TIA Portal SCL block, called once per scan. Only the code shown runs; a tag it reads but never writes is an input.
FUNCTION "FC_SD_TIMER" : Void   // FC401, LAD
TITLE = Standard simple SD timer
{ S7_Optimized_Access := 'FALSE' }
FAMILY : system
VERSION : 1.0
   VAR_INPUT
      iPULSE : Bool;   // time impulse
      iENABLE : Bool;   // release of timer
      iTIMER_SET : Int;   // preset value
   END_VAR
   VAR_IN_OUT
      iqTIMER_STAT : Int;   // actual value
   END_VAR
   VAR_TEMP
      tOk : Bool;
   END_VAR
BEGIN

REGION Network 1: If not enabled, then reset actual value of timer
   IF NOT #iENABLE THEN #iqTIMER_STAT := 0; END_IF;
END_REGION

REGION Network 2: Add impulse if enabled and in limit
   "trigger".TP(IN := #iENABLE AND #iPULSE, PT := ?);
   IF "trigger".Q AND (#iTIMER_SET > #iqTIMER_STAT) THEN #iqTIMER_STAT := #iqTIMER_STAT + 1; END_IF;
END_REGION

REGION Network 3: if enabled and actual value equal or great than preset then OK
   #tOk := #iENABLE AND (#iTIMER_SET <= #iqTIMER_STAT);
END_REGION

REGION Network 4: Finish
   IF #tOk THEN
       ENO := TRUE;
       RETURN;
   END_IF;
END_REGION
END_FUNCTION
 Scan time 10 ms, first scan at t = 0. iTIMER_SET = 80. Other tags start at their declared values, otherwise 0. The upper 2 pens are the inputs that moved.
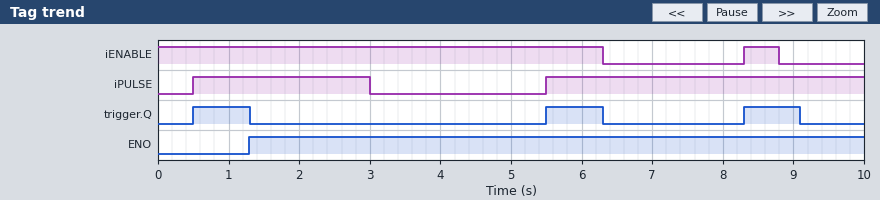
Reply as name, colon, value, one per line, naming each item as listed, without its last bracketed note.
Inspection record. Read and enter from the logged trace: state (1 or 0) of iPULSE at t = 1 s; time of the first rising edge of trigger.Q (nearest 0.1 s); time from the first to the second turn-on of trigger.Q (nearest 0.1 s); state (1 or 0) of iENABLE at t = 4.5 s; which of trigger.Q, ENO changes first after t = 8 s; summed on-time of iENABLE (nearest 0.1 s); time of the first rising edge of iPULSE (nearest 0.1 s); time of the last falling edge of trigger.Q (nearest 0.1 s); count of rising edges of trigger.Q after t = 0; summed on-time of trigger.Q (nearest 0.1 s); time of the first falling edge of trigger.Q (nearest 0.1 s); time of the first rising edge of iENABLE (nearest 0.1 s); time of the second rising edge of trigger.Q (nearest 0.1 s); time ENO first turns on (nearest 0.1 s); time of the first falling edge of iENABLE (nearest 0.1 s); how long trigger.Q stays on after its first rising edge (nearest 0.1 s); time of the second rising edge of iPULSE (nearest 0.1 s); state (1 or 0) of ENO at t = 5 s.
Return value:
state (1 or 0) of iPULSE at t = 1 s: 1
time of the first rising edge of trigger.Q: 0.5 s
time from the first to the second turn-on of trigger.Q: 5.0 s
state (1 or 0) of iENABLE at t = 4.5 s: 1
which of trigger.Q, ENO changes first after t = 8 s: trigger.Q
summed on-time of iENABLE: 6.8 s
time of the first rising edge of iPULSE: 0.5 s
time of the last falling edge of trigger.Q: 9.1 s
count of rising edges of trigger.Q after t = 0: 3
summed on-time of trigger.Q: 2.4 s
time of the first falling edge of trigger.Q: 1.3 s
time of the first rising edge of iENABLE: 8.3 s
time of the second rising edge of trigger.Q: 5.5 s
time ENO first turns on: 1.3 s
time of the first falling edge of iENABLE: 6.3 s
how long trigger.Q stays on after its first rising edge: 0.8 s
time of the second rising edge of iPULSE: 5.5 s
state (1 or 0) of ENO at t = 5 s: 1
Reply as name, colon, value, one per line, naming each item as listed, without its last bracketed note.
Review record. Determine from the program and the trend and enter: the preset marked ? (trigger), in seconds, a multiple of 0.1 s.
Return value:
the preset marked ? (trigger), in seconds, a multiple of 0.1 s: 0.8 s
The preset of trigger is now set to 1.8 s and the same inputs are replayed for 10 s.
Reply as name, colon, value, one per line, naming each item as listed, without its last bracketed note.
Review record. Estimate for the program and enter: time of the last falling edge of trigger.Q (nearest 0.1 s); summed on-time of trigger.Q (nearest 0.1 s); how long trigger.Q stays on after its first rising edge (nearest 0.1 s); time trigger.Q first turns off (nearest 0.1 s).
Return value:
time of the last falling edge of trigger.Q: 7.3 s
summed on-time of trigger.Q: 5.3 s
how long trigger.Q stays on after its first rising edge: 1.8 s
time trigger.Q first turns off: 2.3 s
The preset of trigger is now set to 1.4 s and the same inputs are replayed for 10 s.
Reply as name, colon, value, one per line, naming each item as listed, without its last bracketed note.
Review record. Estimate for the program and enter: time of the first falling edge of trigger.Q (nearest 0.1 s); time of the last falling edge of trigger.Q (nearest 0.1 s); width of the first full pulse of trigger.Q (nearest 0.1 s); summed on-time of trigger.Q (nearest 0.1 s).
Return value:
time of the first falling edge of trigger.Q: 1.9 s
time of the last falling edge of trigger.Q: 9.7 s
width of the first full pulse of trigger.Q: 1.4 s
summed on-time of trigger.Q: 4.2 s
